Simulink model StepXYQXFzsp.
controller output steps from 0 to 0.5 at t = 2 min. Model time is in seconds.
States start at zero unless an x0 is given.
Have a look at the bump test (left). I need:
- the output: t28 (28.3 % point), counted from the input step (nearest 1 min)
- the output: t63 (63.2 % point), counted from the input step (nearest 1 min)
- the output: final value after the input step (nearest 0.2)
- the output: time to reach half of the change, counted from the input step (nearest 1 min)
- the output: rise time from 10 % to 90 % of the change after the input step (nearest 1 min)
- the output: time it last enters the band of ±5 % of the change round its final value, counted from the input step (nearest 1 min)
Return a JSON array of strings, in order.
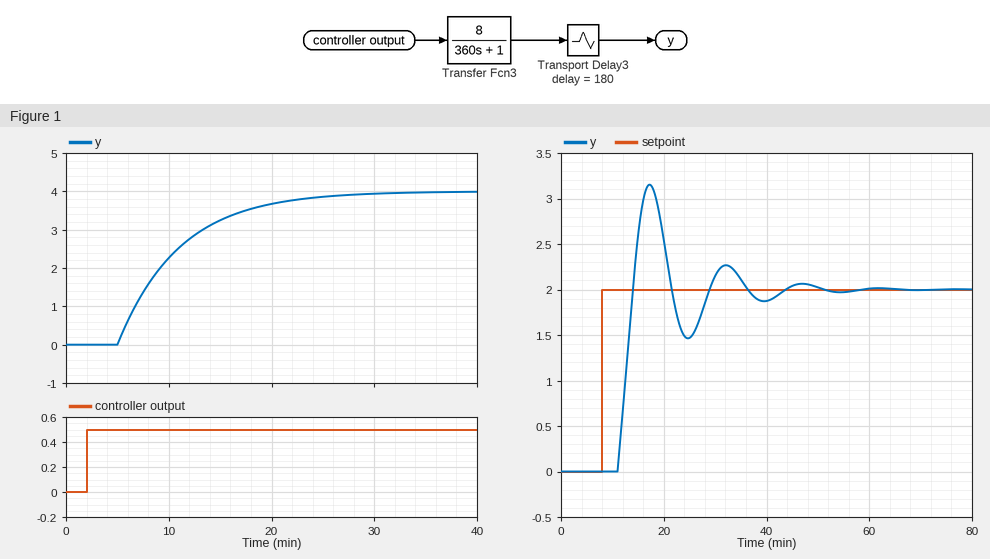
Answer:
["5 min", "9 min", "4.0", "7 min", "13 min", "21 min"]
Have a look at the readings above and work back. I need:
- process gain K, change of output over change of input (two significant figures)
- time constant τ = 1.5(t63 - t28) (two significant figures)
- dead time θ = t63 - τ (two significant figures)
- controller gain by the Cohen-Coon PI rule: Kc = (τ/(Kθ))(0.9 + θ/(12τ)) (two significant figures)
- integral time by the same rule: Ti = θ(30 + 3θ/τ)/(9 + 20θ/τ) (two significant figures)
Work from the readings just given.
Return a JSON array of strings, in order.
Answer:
["8.0", "6.0 min", "3.0 min", "0.24", "5.0 min"]
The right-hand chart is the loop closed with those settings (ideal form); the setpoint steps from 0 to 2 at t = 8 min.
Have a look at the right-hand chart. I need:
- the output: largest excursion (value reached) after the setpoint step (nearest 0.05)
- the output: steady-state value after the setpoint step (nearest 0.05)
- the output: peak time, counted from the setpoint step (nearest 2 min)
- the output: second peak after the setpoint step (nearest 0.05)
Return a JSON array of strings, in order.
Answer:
["3.15", "2.00", "10 min", "2.25"]
